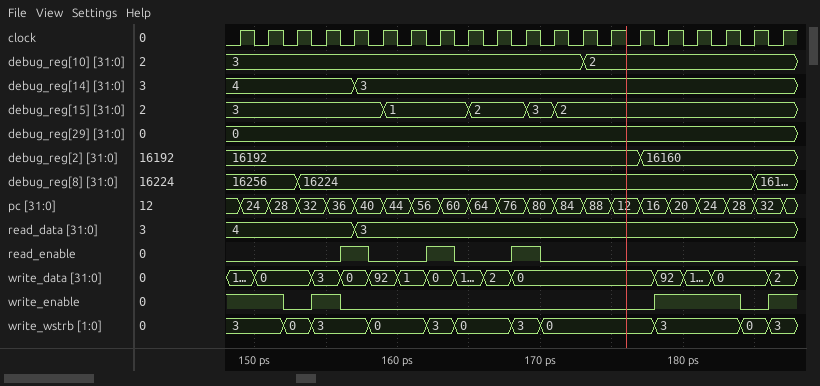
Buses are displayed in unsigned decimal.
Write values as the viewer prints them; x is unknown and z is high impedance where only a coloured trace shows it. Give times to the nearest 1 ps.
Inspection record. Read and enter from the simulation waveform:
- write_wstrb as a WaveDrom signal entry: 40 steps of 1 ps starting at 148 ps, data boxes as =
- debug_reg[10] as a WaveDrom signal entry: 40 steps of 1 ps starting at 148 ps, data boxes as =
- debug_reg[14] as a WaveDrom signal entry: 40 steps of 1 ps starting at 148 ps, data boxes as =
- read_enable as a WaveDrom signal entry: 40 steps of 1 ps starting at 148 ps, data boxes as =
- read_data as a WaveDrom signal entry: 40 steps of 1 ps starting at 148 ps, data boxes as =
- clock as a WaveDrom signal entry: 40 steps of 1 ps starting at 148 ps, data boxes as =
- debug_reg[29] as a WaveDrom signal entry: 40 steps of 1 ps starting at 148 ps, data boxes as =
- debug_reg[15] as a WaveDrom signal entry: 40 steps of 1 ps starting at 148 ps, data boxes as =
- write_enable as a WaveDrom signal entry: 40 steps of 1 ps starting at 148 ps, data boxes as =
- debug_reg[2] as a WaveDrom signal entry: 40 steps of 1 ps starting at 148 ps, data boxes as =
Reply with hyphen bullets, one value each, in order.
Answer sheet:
- {name: 'write_wstrb', wave: '=...=.=...=...=.=...=.=.......=.....=.=.', data: '3 0 3 0 3 0 3 0 3 0 3'}
- {name: 'debug_reg[10]', wave: '=........................=..............', data: '3 2'}
- {name: 'debug_reg[14]', wave: '=........=..............................', data: '4 3'}
- {name: 'read_enable', wave: '0.......1.0...1.0...1.0.................'}
- {name: 'read_data', wave: '=........=..............................', data: '4 3'}
- {name: 'clock', wave: '0101010101010101010101010101010101010101'}
- {name: 'debug_reg[29]', wave: '=.......................................', data: '0'}
- {name: 'debug_reg[15]', wave: '=..........=.....=...=.=................', data: '3 1 2 3 2'}
- {name: 'write_enable', wave: '1...0.1.0.....................1.....0.1.'}
- {name: 'debug_reg[2]', wave: '=............................=..........', data: '16192 16160'}
